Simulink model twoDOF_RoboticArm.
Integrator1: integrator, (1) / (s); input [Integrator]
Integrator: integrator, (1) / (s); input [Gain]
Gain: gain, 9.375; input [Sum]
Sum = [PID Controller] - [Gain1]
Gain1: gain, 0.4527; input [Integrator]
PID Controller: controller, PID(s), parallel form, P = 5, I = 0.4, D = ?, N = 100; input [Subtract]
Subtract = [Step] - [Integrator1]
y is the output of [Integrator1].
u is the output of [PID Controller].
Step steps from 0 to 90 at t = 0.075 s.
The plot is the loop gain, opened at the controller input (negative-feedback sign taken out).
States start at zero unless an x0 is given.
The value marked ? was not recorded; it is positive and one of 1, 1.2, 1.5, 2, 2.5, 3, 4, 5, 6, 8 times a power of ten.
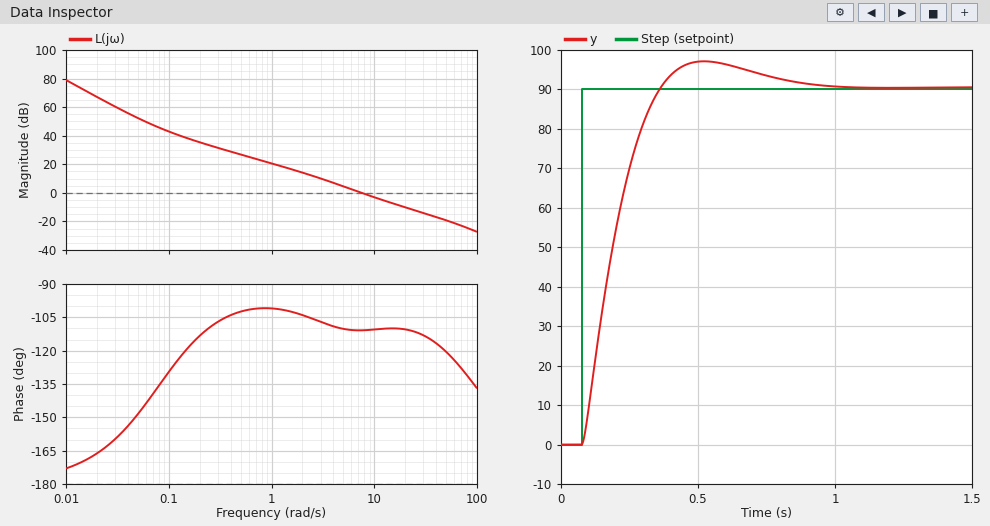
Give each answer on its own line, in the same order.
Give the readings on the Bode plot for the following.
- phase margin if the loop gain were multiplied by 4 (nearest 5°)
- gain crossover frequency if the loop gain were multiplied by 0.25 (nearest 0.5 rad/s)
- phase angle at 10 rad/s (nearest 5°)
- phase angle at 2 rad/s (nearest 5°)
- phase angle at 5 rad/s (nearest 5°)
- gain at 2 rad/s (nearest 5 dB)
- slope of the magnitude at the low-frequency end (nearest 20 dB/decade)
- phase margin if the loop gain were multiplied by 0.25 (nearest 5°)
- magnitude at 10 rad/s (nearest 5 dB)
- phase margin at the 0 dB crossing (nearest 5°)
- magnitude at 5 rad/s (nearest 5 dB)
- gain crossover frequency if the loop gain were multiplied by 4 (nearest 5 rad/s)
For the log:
70°
2.5 rad/s
-110°
-105°
-110°
15 dB
-40 dB/decade
75°
-5 dB
70°
5 dB
25 rad/s
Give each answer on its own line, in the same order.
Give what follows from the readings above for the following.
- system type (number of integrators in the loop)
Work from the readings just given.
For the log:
2
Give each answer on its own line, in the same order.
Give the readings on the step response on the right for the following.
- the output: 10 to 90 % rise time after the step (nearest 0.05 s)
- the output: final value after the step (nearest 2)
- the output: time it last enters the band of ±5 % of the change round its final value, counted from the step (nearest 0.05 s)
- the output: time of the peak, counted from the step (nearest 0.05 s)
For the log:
0.20 s
90
0.60 s
0.45 s
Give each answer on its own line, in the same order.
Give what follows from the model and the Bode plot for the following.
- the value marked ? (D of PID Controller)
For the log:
0.6
